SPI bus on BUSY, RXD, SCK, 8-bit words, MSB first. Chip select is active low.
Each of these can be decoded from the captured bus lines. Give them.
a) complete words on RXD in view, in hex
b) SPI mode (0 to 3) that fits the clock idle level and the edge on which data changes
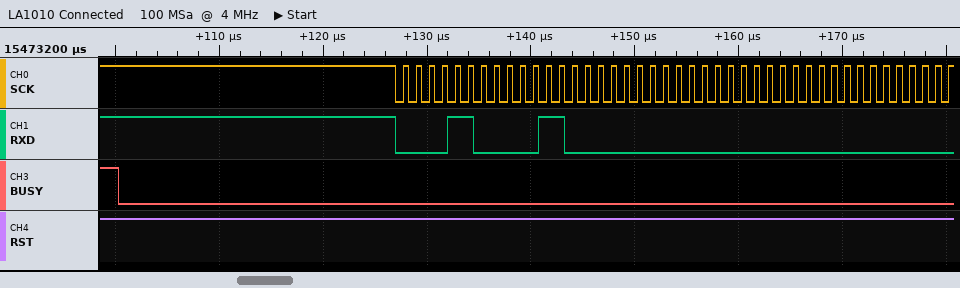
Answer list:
0C, 18, 00, 00, 00
3
